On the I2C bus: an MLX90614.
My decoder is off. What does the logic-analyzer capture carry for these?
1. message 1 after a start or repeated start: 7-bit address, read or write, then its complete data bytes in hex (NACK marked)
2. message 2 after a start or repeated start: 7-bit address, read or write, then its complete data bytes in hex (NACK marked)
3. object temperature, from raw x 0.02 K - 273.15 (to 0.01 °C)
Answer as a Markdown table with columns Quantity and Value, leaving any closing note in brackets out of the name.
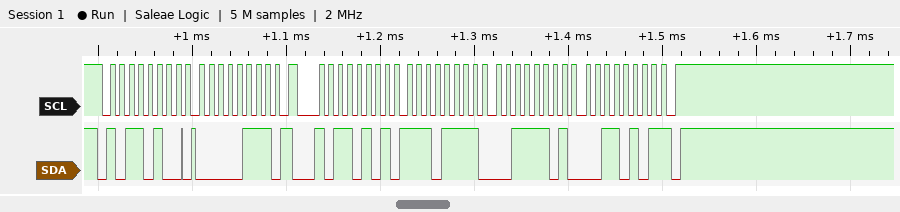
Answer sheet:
| Quantity | Value |
|---|---|
| message 1 after a start or repeated start: 7-bit address, read or write, then its complete data bytes in hex | 0x5A write: 07 |
| message 2 after a start or repeated start: 7-bit address, read or write, then its complete data bytes in hex | 0x5A read: EF 3D 35 NACK |
| object temperature, from raw x 0.02 K - 273.15 | 43.95 °C |
